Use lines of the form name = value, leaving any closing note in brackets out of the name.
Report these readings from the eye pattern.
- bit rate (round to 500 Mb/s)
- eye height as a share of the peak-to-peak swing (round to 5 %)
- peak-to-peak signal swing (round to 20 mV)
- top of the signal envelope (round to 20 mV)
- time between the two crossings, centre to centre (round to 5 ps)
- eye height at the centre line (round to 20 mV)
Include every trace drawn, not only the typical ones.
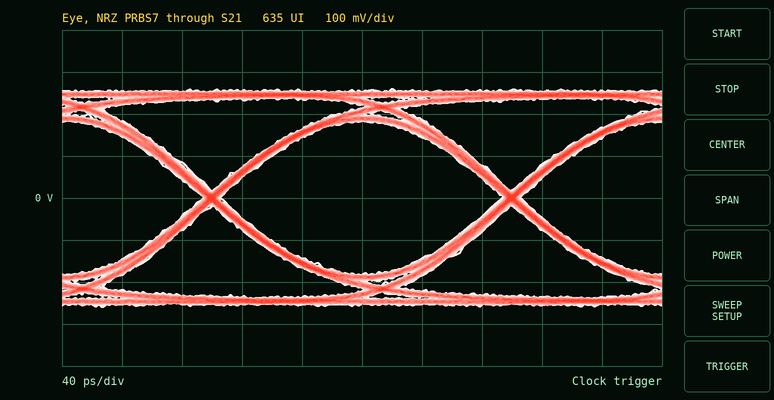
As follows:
bit rate = 5.0 Gb/s
eye height as a share of the peak-to-peak swing = 70 %
peak-to-peak signal swing = 520 mV
top of the signal envelope = 260 mV
time between the two crossings, centre to centre = 200 ps
eye height at the centre line = 360 mV
